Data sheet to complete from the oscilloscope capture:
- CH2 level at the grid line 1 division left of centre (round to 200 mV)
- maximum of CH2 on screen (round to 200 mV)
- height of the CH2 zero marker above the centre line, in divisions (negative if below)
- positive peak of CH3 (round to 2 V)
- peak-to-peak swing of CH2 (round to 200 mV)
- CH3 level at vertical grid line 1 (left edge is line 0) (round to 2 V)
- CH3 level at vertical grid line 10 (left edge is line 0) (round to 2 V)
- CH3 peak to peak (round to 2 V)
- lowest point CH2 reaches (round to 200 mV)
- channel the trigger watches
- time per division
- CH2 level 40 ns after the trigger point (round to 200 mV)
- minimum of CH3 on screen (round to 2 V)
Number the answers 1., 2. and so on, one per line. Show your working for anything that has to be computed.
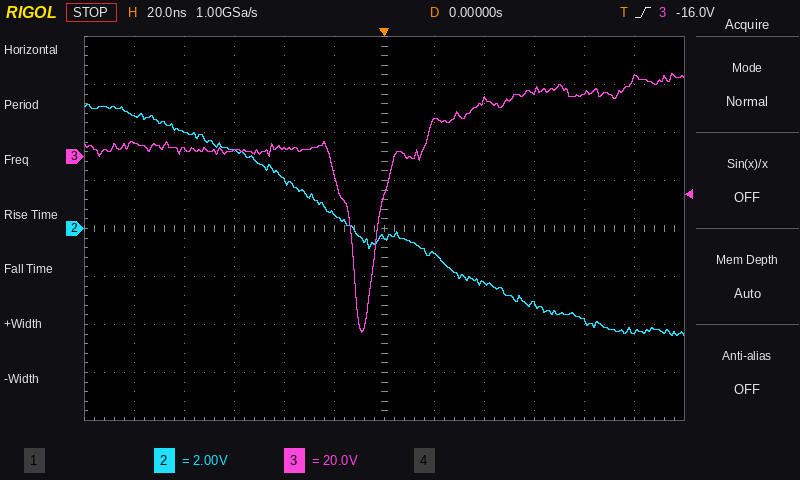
1. 600 mV
2. 5.2 V
3. 0.0 div
4. 34 V
5. 5.2 V − (-4.4 V) = 9.6 V
6. 6 V
7. 26 V
8. 34 V − (-74 V) = 108 V
9. -4.4 V
10. CH3
11. 20 ns
12. -2.2 V
13. -74 V
